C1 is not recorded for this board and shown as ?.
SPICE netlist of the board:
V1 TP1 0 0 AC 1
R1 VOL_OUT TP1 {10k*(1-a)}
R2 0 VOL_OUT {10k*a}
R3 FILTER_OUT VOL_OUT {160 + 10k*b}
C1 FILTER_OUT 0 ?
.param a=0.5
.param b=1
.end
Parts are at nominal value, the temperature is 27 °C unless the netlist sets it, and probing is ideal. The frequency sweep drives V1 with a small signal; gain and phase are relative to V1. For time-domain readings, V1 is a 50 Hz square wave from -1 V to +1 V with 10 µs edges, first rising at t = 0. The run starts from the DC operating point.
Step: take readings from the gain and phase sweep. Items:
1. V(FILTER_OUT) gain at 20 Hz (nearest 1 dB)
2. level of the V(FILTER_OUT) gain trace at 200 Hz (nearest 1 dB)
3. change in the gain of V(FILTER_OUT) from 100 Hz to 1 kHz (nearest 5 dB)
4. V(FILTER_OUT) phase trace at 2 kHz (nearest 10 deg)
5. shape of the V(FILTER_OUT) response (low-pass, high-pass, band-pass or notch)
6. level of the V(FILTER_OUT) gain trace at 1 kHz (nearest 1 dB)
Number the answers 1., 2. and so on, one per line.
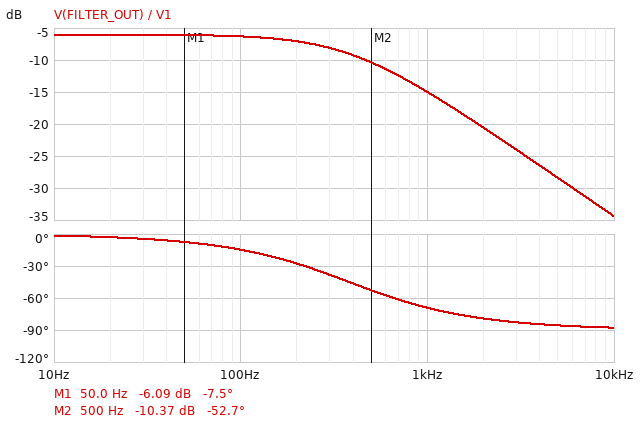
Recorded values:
1. -6 dB
2. -7 dB
3. -10 dB
4. -80 deg
5. low-pass
6. -15 dB
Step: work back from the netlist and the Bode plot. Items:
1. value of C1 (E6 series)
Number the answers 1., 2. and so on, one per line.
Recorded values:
1. 33 nF
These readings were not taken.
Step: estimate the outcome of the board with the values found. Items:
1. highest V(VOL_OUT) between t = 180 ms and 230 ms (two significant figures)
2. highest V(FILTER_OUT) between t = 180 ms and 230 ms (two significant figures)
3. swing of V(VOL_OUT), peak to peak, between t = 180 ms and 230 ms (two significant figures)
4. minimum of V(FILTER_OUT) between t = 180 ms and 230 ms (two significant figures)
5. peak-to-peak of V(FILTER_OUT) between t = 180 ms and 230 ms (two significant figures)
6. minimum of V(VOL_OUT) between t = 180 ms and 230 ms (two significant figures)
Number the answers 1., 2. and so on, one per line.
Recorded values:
1. 500 mV
2. 500 mV
3. 1.0 V
4. -500 mV
5. 1.0 V
6. -500 mV
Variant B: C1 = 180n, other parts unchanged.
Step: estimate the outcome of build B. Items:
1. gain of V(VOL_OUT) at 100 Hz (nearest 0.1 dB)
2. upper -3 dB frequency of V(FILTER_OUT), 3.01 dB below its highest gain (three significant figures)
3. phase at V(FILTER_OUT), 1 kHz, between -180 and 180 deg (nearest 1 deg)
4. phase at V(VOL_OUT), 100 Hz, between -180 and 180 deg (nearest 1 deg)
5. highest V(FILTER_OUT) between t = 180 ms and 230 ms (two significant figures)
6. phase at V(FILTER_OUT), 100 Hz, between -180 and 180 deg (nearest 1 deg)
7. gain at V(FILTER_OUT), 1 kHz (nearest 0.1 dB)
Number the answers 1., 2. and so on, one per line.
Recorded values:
1. -7.2 dB
2. 69.8 Hz
3. -86 deg
4. -6 deg
5. 490 mV
6. -55 deg
7. -29.2 dB
